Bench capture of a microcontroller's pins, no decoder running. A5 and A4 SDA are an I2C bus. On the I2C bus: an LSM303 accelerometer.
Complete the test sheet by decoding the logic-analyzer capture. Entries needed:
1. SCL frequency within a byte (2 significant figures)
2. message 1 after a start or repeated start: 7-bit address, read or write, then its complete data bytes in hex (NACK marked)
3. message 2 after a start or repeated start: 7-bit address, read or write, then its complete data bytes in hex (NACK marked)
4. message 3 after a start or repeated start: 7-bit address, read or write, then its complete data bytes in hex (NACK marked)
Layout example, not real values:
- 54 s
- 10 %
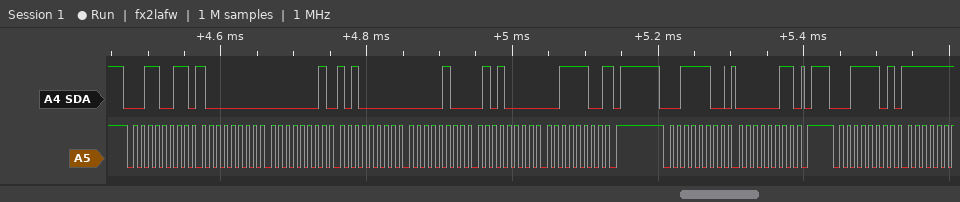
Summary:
- 100 kHz
- 0x19 read: 80 01 A0 04 50 3C NACK
- 0x1E write: 03
- 0x1E read
